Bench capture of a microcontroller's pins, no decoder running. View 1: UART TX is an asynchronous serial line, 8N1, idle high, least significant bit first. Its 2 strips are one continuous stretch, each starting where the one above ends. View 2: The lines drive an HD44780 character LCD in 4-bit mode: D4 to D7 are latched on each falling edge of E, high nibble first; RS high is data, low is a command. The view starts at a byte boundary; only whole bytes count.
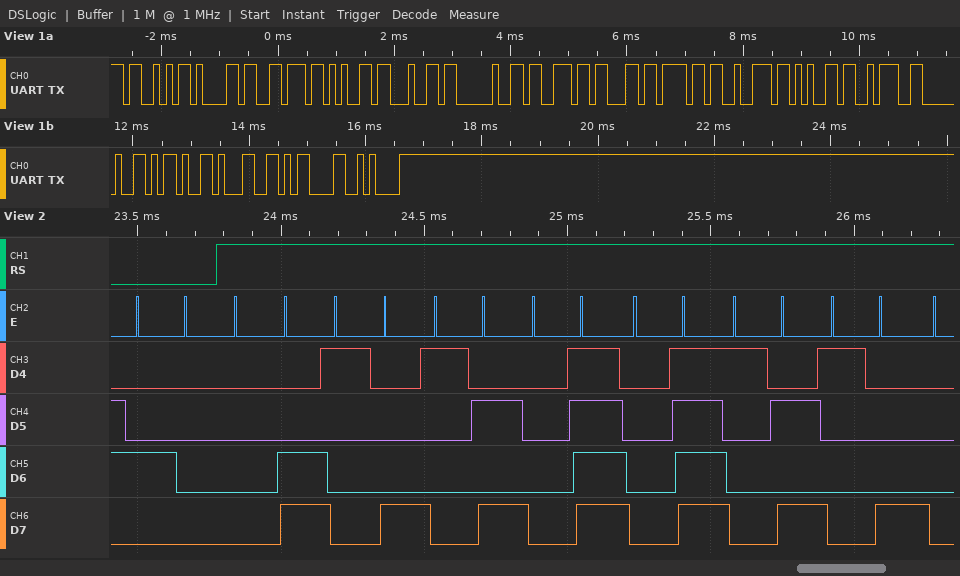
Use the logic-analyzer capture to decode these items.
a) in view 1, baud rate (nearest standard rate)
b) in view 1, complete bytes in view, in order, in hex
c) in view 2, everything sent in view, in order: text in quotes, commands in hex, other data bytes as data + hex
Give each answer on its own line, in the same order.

9600 baud
0x53 0x61 0x76 0x65 0x64 0x20 0x73 0x63 0x6F 0x72 0x65 0x3A 0x20 0x2D 0x31 0x0D 0x0A
0x40 data 0C 18 1A 0F 0F 1A 18
